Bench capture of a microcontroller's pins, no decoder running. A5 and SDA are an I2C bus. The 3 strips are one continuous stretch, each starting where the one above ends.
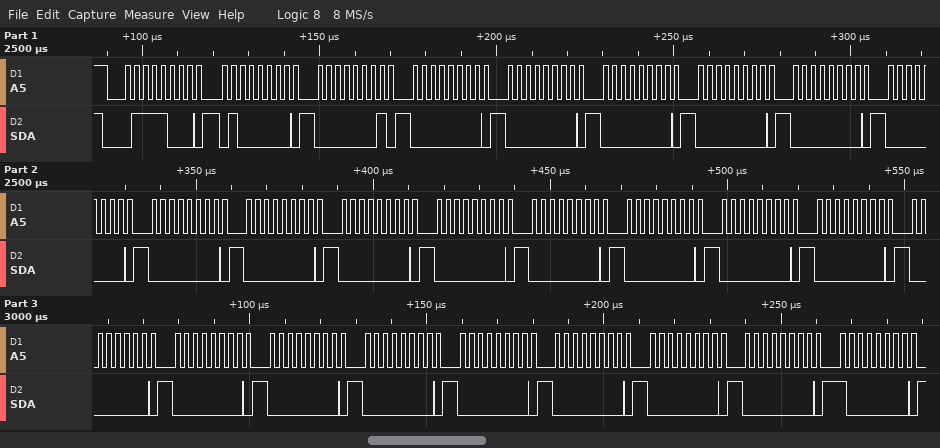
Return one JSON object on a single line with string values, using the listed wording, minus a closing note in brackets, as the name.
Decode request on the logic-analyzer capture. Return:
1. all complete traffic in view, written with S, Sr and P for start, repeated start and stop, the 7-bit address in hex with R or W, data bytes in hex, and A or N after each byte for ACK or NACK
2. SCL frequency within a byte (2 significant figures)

{"all complete traffic in view, written with S, Sr and P for start, repeated start and stop, the 7-bit address in hex with R or W, data bytes in hex, and A or N after each byte for ACK or NACK": "S 3CW A 40 A 01 A 00 A 00 A 00 A 00 A 00 A 00 A 00 A 00 A 00 A 00 A 00 A 00 A 00 A 00 A 00 A 00 A 00 A 00 A 00 A 00 A 00 A 00 A 80 A", "SCL frequency within a byte": "400 kHz"}
